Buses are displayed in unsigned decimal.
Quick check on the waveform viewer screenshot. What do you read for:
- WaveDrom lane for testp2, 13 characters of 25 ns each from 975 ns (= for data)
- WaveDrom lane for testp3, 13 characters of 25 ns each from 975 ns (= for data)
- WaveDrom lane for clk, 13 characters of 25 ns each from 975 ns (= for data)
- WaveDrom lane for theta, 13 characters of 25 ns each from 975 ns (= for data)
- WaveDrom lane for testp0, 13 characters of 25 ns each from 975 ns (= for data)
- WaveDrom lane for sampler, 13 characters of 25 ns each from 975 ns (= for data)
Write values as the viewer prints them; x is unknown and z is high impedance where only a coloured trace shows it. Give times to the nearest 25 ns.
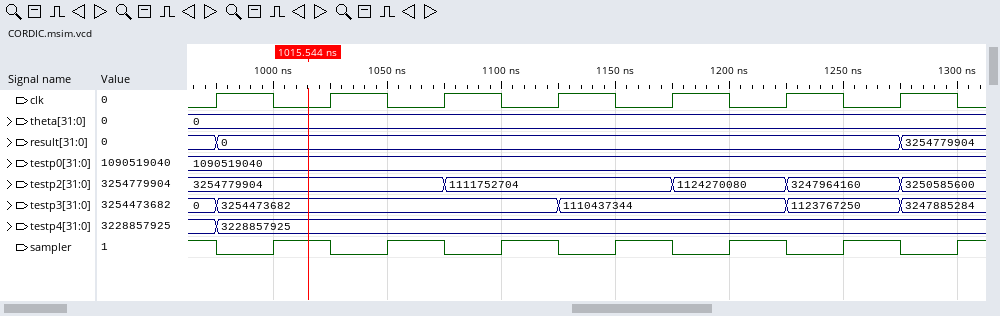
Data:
{name: 'testp2', wave: '=...=...=.=.=', data: '3254779904 1111752704 1124270080 3247964160 3250585600'}
{name: 'testp3', wave: '=.....=...=.=', data: '3254473682 1110437344 1123767250 3247885284'}
{name: 'clk', wave: '1010101010101'}
{name: 'theta', wave: '=............', data: '0'}
{name: 'testp0', wave: '=............', data: '1090519040'}
{name: 'sampler', wave: '0101010101010'}
